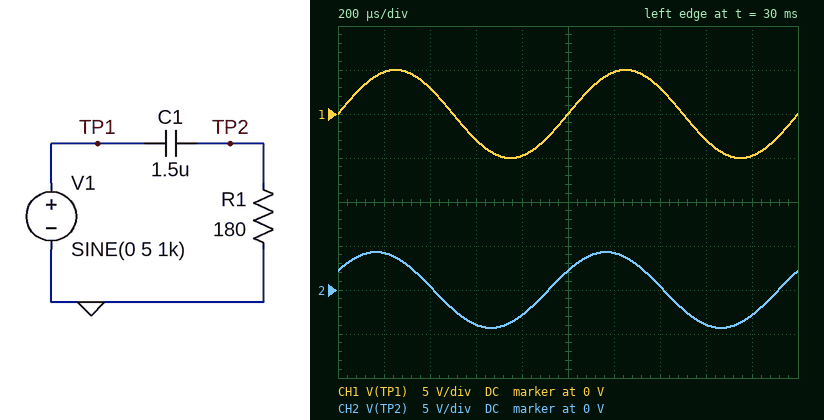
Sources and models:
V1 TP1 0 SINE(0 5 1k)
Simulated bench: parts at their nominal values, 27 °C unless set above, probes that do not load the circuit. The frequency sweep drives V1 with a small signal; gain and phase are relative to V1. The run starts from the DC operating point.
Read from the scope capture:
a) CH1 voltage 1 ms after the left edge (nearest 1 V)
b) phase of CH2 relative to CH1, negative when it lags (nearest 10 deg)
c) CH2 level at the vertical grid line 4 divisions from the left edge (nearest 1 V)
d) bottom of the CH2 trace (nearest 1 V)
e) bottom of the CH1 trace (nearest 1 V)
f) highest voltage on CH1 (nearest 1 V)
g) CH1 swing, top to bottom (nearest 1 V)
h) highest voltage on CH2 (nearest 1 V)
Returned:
0 V
30 deg
-3 V
-4 V
-5 V
5 V
10 V
4 V
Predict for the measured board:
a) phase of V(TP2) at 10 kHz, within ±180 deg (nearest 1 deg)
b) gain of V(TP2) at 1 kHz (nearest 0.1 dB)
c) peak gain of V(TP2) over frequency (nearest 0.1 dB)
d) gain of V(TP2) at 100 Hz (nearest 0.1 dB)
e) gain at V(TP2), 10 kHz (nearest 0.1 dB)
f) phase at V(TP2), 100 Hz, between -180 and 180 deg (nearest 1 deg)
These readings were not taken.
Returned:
3 deg
-1.3 dB
0 dB
-15.5 dB
0 dB
80 deg
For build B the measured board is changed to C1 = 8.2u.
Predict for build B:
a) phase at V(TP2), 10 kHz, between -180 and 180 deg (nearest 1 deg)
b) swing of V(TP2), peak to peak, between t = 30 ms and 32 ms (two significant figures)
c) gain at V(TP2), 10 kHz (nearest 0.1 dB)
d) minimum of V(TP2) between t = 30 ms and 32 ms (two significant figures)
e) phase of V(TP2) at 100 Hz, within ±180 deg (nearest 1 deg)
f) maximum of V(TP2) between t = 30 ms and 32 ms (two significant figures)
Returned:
1 deg
9.9 V
0 dB
-5.0 V
47 deg
5.0 V
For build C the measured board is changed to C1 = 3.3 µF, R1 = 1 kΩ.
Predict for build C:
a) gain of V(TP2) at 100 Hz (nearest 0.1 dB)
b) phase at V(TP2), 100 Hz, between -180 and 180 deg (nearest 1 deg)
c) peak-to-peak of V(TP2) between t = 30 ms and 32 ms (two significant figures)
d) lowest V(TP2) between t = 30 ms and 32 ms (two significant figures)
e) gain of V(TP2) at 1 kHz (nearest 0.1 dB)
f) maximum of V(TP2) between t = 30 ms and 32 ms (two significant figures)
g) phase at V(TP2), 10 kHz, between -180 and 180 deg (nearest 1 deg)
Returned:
-0.9 dB
26 deg
10 V
-5.0 V
0 dB
5.0 V
0 deg
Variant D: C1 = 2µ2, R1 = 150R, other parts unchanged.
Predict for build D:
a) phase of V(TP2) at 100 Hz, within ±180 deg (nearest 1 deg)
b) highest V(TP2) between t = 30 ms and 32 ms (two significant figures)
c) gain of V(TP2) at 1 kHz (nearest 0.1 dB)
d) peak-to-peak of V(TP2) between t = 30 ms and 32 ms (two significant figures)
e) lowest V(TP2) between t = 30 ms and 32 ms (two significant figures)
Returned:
78 deg
4.5 V
-0.9 dB
9.0 V
-4.5 V
